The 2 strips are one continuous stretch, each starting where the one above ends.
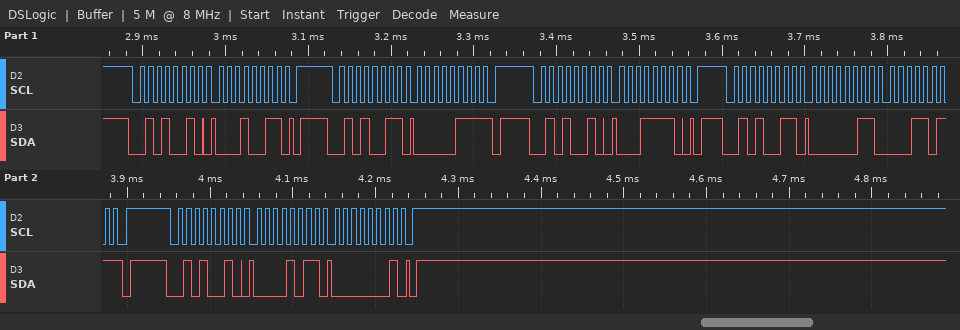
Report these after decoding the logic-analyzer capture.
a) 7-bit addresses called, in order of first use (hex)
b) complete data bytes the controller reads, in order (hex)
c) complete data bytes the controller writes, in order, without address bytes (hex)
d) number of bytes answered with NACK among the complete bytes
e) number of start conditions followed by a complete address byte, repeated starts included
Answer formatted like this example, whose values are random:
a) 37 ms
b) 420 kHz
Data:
a) 0x29
b) 07 03 1B
c) 13 1E 0B 01
d) 2
e) 5
